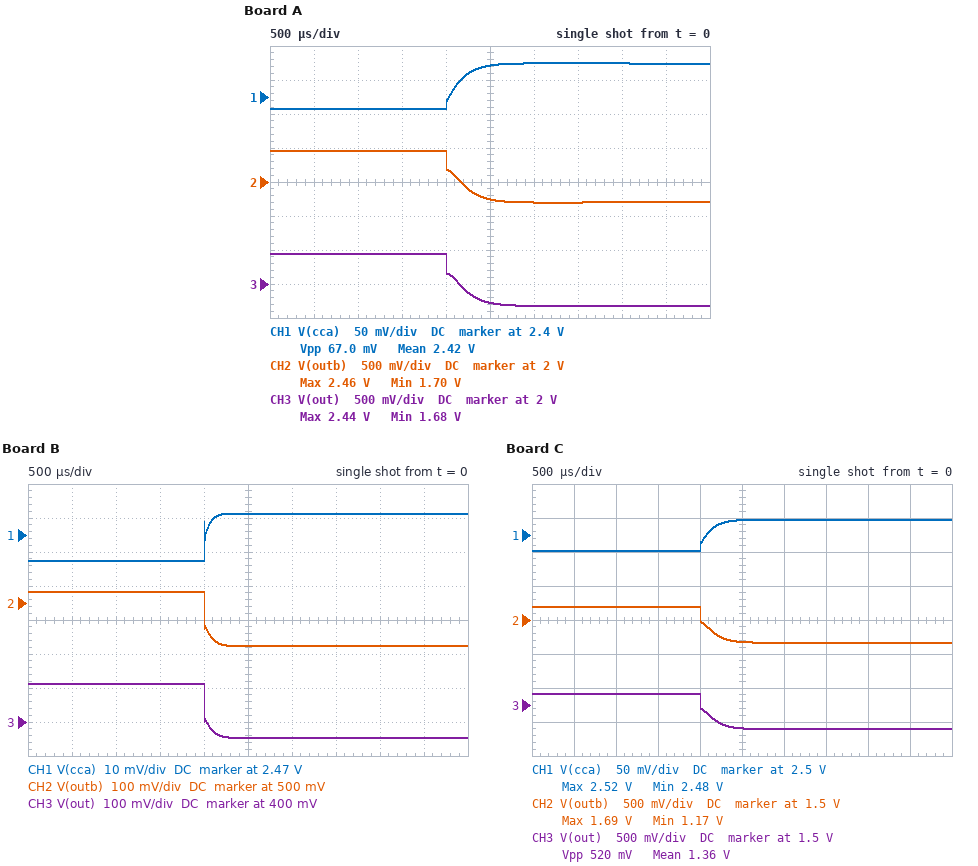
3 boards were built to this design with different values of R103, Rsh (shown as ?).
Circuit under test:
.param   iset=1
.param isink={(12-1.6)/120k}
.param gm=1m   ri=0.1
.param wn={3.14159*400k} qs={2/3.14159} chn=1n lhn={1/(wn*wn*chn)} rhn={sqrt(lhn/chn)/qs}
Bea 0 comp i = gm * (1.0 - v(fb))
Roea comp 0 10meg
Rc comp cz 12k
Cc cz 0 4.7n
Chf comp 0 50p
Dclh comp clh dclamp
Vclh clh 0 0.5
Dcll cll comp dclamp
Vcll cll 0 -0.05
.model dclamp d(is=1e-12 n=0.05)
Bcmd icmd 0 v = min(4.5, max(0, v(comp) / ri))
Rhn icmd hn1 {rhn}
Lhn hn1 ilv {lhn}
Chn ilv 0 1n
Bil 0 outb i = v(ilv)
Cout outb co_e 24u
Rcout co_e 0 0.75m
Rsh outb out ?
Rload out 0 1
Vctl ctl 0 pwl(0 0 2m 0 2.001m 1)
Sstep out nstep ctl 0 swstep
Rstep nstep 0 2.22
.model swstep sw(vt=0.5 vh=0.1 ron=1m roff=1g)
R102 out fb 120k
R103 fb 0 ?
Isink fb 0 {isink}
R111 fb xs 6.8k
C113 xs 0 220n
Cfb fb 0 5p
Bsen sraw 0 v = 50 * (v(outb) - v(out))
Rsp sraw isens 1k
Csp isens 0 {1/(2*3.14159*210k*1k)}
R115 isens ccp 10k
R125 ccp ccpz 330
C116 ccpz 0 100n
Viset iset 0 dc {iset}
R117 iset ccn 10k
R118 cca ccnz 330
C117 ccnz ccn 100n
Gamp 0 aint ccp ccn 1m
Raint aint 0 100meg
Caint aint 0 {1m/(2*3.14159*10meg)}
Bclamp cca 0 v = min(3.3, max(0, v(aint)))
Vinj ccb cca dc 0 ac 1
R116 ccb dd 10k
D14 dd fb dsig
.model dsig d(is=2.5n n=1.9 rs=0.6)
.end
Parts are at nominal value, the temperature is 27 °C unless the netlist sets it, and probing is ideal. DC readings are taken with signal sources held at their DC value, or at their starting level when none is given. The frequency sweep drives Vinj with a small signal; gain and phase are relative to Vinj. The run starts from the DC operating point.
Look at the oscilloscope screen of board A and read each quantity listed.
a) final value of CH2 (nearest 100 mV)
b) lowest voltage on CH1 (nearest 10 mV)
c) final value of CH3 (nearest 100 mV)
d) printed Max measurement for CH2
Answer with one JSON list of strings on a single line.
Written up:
["1.7 V", "2.38 V", "1.7 V", "2.46 V"]
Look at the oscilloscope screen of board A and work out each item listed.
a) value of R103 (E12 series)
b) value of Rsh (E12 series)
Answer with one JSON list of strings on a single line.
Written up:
["82 kΩ", "8.2 mΩ"]
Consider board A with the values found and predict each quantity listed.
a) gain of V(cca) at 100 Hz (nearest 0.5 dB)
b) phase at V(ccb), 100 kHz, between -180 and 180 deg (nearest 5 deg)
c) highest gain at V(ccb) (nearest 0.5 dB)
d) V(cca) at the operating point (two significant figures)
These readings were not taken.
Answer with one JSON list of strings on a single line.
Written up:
["0 dB", "0 deg", "0.5 dB", "2.4 V"]
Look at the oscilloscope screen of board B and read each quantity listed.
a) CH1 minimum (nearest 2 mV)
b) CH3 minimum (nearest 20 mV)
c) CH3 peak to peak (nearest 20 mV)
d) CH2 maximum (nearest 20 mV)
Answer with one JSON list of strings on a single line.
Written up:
["2.462 V", "360 mV", "160 mV", "540 mV"]
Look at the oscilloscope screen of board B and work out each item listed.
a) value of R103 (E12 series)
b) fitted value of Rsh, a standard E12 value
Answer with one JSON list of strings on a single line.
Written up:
["270 kΩ", "0.039 Ω"]
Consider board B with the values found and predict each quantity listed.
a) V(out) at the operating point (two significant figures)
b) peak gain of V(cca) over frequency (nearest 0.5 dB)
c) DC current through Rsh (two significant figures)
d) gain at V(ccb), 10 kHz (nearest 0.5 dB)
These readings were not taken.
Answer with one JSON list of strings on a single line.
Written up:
["510 mV", "0 dB", "510 mA", "-3.5 dB"]
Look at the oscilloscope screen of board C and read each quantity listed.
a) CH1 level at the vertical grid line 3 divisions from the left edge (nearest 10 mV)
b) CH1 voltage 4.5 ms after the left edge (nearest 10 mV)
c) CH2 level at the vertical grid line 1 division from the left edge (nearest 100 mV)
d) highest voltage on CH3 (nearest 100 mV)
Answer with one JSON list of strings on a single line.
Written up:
["2.48 V", "2.52 V", "1.7 V", "1.7 V"]
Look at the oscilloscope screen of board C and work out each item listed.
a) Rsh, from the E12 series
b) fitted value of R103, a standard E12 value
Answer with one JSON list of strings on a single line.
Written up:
["0.012 Ω", "68 kΩ"]
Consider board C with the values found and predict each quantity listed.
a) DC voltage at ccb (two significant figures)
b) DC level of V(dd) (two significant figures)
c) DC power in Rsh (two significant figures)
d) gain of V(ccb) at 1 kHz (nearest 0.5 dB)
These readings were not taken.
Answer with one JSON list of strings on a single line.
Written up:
["2.5 V", "1.5 V", "33 mW", "-3.5 dB"]
